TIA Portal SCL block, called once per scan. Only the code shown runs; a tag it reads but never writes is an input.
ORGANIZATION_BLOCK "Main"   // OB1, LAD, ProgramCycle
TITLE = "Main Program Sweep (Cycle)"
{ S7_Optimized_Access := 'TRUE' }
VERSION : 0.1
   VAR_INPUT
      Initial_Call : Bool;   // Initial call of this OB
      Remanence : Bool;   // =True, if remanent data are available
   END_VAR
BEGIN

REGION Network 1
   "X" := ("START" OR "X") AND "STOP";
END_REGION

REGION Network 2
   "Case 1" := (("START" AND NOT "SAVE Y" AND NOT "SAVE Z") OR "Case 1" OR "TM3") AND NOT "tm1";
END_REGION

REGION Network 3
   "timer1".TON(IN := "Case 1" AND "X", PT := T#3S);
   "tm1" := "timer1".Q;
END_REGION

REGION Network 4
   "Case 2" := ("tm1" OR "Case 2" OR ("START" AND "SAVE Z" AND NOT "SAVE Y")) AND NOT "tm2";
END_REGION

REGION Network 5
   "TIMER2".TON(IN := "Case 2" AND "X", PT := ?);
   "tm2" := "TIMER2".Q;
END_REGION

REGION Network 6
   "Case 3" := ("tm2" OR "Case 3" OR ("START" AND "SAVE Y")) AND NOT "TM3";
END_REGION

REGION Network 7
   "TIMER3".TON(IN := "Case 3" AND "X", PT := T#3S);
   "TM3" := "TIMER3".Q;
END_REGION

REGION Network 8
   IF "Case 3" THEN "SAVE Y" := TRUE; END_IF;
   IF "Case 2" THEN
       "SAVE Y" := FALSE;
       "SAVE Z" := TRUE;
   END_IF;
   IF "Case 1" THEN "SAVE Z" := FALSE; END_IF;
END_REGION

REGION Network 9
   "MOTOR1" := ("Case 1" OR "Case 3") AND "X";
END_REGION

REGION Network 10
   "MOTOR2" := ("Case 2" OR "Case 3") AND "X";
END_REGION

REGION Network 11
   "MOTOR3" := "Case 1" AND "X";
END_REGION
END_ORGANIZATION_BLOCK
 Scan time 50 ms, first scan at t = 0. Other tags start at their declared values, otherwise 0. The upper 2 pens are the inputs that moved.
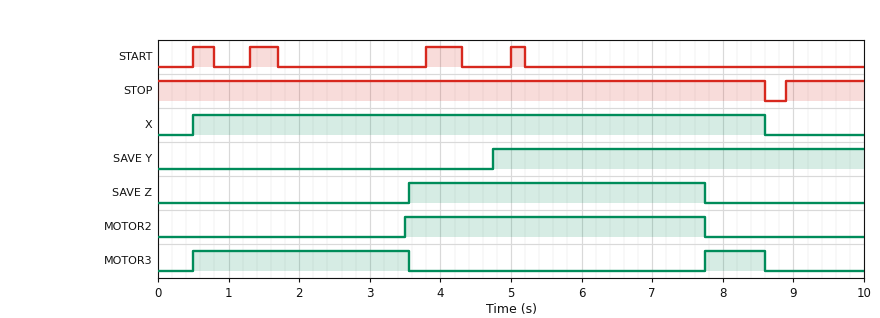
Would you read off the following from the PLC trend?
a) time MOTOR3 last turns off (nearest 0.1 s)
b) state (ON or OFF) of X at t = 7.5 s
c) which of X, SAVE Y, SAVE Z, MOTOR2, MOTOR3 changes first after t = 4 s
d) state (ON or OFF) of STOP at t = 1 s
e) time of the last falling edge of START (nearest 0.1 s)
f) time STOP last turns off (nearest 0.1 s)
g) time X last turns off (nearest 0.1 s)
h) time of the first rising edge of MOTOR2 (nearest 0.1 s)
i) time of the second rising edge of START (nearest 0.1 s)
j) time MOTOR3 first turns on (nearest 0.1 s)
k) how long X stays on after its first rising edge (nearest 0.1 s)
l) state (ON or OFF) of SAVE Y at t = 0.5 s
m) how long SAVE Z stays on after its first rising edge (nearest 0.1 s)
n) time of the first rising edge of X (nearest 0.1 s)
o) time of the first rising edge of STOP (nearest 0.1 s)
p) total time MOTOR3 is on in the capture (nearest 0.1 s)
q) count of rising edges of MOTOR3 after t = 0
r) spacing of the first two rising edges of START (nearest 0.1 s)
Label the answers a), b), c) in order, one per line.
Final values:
a) 8.6 s
b) ON
c) SAVE Y
d) ON
e) 5.2 s
f) 8.6 s
g) 8.6 s
h) 3.5 s
i) 1.3 s
j) 0.5 s
k) 8.1 s
l) OFF
m) 4.2 s
n) 0.5 s
o) 8.9 s
p) 3.9 s
q) 2
r) 0.8 s
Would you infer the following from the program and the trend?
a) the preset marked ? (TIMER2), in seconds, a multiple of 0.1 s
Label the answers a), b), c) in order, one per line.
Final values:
a) 1.2 s
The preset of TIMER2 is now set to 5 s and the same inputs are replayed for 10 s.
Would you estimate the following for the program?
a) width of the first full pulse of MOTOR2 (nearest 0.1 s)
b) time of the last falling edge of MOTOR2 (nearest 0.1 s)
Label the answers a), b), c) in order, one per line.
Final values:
a) 5.1 s
b) 8.6 s
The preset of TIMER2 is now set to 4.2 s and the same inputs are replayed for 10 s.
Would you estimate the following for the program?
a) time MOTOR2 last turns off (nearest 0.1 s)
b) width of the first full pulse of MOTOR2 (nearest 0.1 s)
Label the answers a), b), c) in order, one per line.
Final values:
a) 8.6 s
b) 5.1 s
